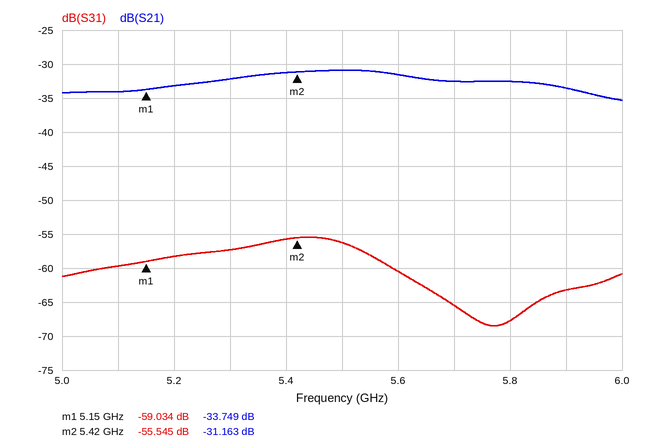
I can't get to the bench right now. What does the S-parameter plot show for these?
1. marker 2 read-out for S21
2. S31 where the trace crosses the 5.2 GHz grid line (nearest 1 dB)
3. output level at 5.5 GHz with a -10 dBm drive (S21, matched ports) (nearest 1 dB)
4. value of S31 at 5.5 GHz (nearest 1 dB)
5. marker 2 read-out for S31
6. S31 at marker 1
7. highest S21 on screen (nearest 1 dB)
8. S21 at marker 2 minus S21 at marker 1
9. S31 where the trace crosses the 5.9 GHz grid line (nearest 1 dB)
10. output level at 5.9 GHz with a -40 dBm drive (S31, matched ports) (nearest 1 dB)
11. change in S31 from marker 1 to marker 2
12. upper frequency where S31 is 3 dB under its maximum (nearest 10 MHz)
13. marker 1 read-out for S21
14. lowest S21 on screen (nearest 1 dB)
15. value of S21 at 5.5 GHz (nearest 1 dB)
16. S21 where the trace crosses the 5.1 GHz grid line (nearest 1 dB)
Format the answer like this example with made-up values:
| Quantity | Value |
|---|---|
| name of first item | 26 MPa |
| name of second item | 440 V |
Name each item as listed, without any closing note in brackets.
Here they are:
| Quantity | Value |
|---|---|
| marker 2 read-out for S21 | -31.163 dB |
| S31 where the trace crosses the 5.2 GHz grid line | -58 dB |
| output level at 5.5 GHz with a -10 dBm drive (S21, matched ports) | -41 dBm |
| value of S31 at 5.5 GHz | -56 dB |
| marker 2 read-out for S31 | -55.545 dB |
| S31 at marker 1 | -59.034 dB |
| highest S21 on screen | -31 dB |
| S21 at marker 2 minus S21 at marker 1 | 2.586 dB |
| S31 where the trace crosses the 5.9 GHz grid line | -63 dB |
| output level at 5.9 GHz with a -40 dBm drive (S31, matched ports) | -103 dBm |
| change in S31 from marker 1 to marker 2 | 3.489 dB |
| upper frequency where S31 is 3 dB under its maximum | 5.56 GHz |
| marker 1 read-out for S21 | -33.749 dB |
| lowest S21 on screen | -35 dB |
| value of S21 at 5.5 GHz | -31 dB |
| S21 where the trace crosses the 5.1 GHz grid line | -34 dB |
